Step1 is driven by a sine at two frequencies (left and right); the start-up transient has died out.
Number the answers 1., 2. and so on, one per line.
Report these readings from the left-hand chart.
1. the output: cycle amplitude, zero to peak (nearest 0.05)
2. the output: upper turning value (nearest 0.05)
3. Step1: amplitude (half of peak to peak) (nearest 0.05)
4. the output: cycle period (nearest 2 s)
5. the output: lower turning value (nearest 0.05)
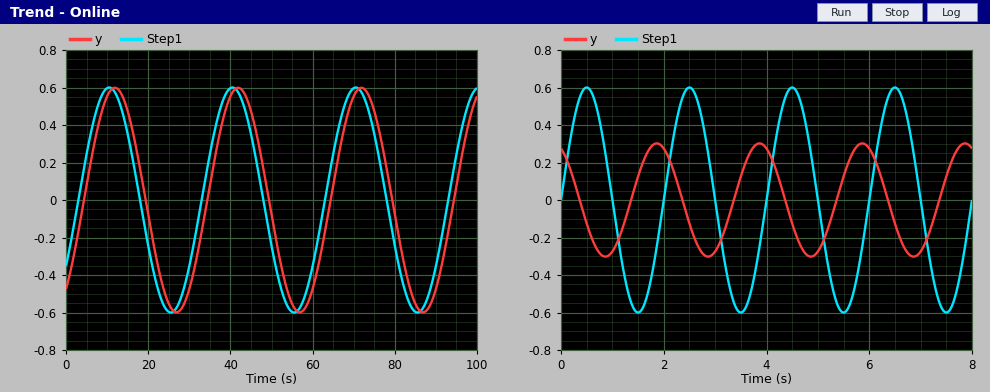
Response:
1. 0.60
2. 0.60
3. 0.60
4. 30 s
5. -0.60
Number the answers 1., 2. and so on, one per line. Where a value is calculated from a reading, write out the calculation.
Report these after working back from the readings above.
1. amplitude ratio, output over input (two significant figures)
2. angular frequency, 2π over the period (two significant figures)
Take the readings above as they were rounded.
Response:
1. 0.6 / 0.6 = 1.0
2. 2π / 30 = 0.21 rad/s
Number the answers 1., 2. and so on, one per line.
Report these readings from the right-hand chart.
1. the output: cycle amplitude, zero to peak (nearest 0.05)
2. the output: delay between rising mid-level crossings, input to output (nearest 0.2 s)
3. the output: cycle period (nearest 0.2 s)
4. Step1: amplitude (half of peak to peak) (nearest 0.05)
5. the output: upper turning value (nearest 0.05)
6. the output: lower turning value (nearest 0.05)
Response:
1. 0.30
2. 1.4 s
3. 2.0 s
4. 0.60
5. 0.30
6. -0.30
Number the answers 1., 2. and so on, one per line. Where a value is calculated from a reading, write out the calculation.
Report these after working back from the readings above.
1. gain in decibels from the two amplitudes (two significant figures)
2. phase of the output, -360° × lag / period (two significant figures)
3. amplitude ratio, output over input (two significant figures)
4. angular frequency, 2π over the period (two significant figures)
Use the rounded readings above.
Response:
1. 20 log10(0.3 / 0.6) = -6.0 dB
2. -360 × 1.4 / 2 = -250°
3. 0.3 / 0.6 = 0.50
4. 2π / 2 = 3.1 rad/s
